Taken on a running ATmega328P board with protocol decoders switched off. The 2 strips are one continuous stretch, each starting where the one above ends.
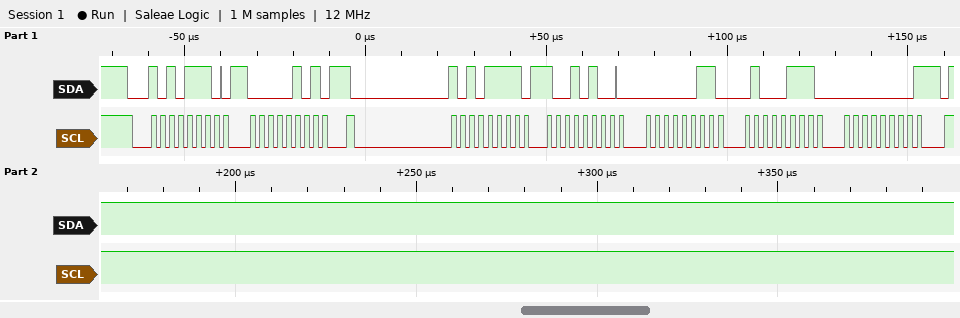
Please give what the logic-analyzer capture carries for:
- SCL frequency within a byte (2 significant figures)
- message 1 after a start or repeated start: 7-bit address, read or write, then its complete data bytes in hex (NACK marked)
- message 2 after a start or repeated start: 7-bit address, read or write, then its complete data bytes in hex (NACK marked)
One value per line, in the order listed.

400 kHz
0x57 write: 05
0x57 read: 94 03 47 00 NACK
